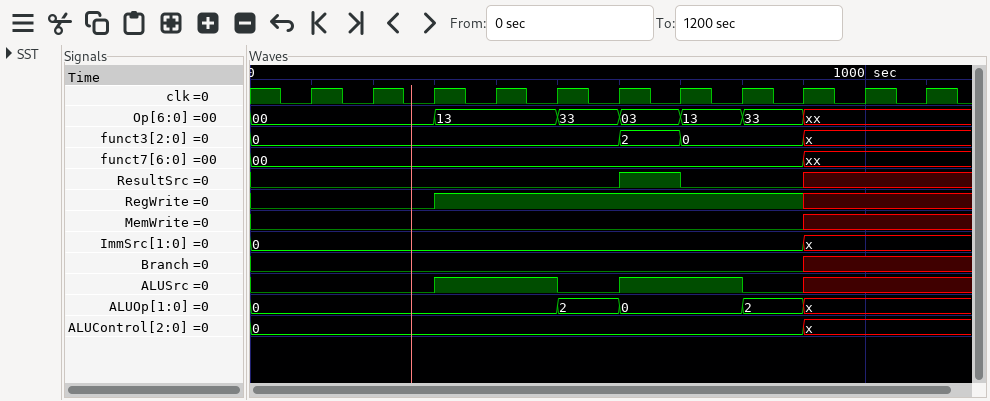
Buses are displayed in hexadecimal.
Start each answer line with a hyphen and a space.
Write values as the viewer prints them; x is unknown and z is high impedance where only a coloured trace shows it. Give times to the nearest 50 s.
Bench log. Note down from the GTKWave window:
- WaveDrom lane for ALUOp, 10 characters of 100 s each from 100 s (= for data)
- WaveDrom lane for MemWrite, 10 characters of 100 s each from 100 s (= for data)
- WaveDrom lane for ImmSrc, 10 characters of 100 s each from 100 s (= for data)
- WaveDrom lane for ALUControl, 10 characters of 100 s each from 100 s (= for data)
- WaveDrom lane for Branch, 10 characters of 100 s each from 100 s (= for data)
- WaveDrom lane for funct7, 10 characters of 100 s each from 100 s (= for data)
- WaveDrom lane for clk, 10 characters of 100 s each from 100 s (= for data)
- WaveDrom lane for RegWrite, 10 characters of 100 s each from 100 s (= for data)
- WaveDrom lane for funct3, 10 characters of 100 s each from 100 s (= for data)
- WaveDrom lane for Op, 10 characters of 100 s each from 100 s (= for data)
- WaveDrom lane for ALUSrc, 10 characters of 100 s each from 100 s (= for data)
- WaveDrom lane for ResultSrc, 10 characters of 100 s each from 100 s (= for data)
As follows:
- {name: 'ALUOp', wave: '=...==.=x.', data: '0 2 0 2'}
- {name: 'MemWrite', wave: '0.......x.'}
- {name: 'ImmSrc', wave: '=.......x.', data: '0'}
- {name: 'ALUControl', wave: '=.......x.', data: '0'}
- {name: 'Branch', wave: '0.......x.'}
- {name: 'funct7', wave: '=.......x.', data: '00'}
- {name: 'clk', wave: 'p.........'}
- {name: 'RegWrite', wave: '0.1.....x.'}
- {name: 'funct3', wave: '=....==.x.', data: '0 2 0'}
- {name: 'Op', wave: '=.=.====x.', data: '00 13 33 03 13 33'}
- {name: 'ALUSrc', wave: '0.1.01.0x.'}
- {name: 'ResultSrc', wave: '0....10.x.'}
